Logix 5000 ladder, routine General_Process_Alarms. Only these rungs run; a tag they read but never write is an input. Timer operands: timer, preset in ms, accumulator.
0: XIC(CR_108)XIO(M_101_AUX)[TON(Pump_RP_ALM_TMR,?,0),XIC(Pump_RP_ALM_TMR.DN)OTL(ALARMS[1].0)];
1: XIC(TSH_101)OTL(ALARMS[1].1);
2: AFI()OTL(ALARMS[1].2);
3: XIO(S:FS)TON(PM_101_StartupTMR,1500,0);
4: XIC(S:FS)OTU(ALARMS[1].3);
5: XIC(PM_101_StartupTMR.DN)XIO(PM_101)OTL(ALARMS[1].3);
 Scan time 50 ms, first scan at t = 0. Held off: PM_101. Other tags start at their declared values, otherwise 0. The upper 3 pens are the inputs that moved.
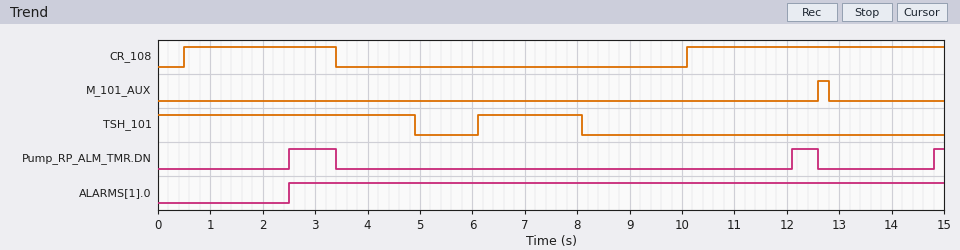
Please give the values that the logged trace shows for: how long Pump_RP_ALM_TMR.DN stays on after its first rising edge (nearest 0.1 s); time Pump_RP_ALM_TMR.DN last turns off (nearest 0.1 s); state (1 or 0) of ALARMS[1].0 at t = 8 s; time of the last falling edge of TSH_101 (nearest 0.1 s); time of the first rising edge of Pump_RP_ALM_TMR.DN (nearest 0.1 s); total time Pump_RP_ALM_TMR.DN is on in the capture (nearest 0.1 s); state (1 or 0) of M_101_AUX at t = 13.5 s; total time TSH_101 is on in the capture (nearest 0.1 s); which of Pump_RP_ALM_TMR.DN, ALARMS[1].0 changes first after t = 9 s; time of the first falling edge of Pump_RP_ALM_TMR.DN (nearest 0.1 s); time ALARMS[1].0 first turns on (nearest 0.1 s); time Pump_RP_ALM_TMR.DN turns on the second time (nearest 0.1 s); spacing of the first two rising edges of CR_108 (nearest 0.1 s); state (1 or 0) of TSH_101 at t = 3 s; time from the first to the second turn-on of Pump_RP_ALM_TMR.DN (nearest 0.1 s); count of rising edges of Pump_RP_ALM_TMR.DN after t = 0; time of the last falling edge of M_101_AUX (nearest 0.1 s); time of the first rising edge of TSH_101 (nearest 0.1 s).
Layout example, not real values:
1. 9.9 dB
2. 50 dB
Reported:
1. 0.9 s
2. 12.6 s
3. 1
4. 8.1 s
5. 2.5 s
6. 1.6 s
7. 0
8. 6.9 s
9. Pump_RP_ALM_TMR.DN
10. 3.4 s
11. 2.5 s
12. 12.1 s
13. 9.6 s
14. 1
15. 9.6 s
16. 3
17. 12.8 s
18. 6.1 s
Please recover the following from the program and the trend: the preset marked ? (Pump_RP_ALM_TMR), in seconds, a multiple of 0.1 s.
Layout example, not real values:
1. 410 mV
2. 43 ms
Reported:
1. 2.0 s
